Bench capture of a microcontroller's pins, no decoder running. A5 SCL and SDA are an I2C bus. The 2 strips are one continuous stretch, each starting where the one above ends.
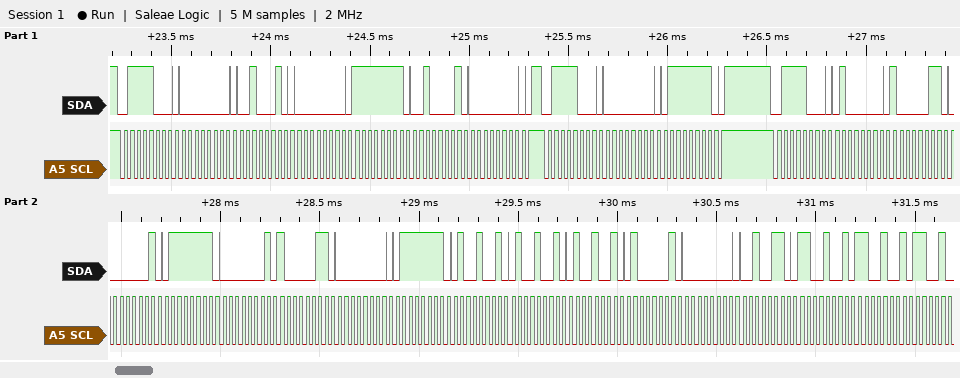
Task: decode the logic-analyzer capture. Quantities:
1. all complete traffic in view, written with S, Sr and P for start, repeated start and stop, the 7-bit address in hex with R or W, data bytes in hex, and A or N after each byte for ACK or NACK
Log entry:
S 3CW A 00 A 22 A 00 A FF A 21 A 00 A P S 3CW A 00 A 7F A P S 3CW A 40 A 83 A 01 A 7F A 01 A 83 A 00 A 7F A 49 A 49 A 49 A 41 A 00 A 26 A C9 A C9 A
